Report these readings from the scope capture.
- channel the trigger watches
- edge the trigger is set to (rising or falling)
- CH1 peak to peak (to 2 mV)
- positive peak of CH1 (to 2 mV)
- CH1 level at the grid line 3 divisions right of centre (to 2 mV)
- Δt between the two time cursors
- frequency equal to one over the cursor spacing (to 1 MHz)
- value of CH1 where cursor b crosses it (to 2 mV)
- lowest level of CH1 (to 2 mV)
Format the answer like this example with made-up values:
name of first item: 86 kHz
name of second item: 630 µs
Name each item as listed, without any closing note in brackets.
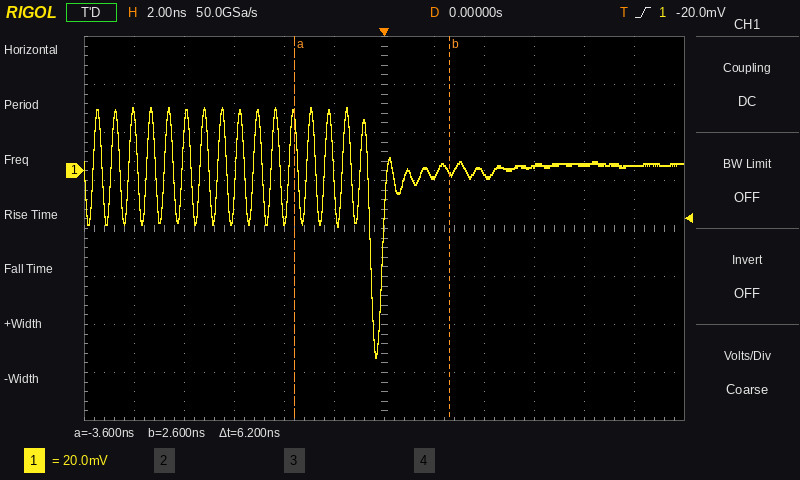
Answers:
channel the trigger watches: CH1
edge the trigger is set to: rising
CH1 peak to peak: 104 mV
positive peak of CH1: 26 mV
CH1 level at the grid line 3 divisions right of centre: 2 mV
Δt between the two time cursors: 6.2 ns
frequency equal to one over the cursor spacing: 161 MHz
value of CH1 where cursor b crosses it: 0 mV
lowest level of CH1: -78 mV
